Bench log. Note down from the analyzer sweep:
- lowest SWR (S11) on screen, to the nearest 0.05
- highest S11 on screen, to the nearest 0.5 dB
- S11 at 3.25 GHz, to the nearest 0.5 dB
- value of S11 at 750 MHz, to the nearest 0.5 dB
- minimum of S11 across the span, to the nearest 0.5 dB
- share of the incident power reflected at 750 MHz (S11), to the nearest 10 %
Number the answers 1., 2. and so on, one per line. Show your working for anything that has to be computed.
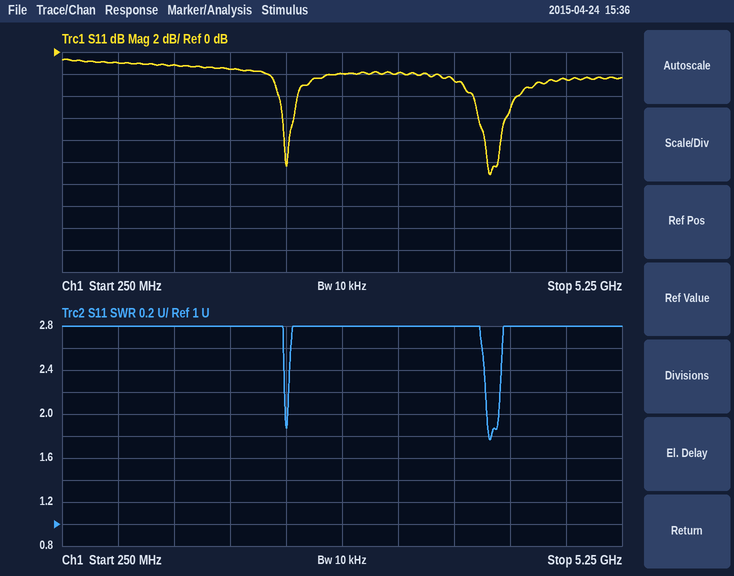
1. 1.75
2. -0.5 dB
3. -2.0 dB
4. -1.0 dB
5. -11.0 dB
6. 10^(-1/10) ≈ 79.4 %, so 80 % to the nearest 10 %
